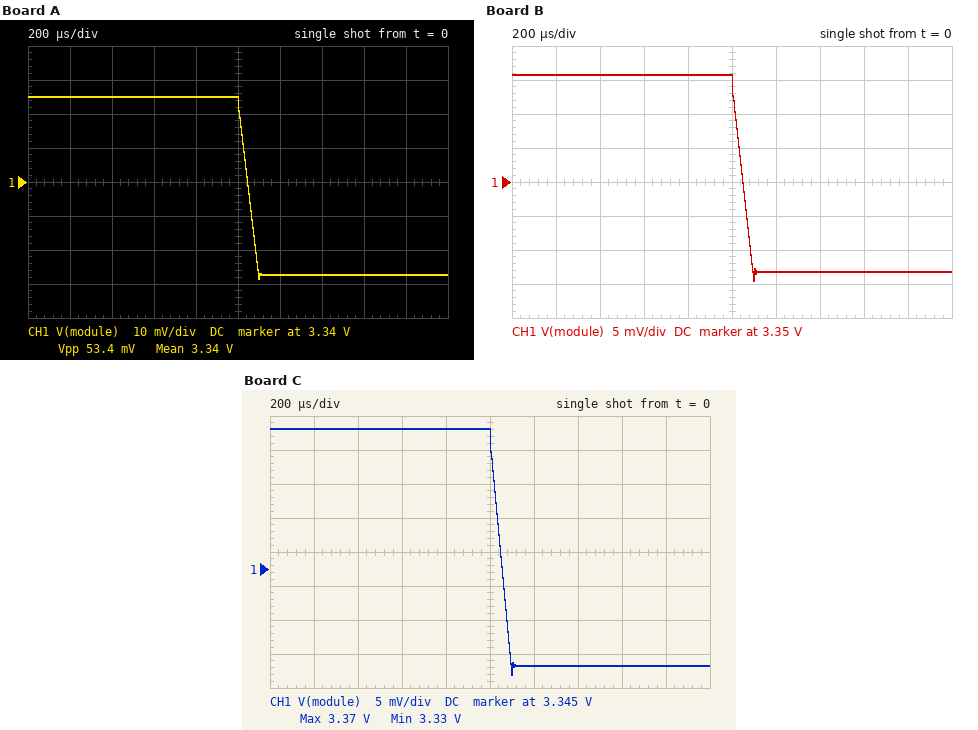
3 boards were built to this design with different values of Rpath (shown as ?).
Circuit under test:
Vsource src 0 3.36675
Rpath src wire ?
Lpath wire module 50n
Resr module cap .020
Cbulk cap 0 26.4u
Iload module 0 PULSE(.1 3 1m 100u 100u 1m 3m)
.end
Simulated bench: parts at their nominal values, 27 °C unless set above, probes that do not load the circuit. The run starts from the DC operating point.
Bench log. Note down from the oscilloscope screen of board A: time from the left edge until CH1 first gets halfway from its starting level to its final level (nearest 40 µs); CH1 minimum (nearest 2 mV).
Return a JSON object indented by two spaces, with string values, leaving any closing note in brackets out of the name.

{
  "time from the left edge until CH1 first gets halfway from its starting level to its final level": "1.04 ms",
  "CH1 minimum": "3.312 V"
}
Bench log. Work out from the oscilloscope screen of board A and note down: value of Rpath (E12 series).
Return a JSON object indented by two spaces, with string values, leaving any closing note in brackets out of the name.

{
  "value of Rpath": "0.018 Ω"
}
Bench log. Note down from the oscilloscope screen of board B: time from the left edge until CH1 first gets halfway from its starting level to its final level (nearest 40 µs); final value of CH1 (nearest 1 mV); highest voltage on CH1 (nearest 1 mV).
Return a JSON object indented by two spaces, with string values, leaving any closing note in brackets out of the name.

{
  "time from the left edge until CH1 first gets halfway from its starting level to its final level": "1.04 ms",
  "final value of CH1": "3.337 V",
  "highest voltage on CH1": "3.366 V"
}
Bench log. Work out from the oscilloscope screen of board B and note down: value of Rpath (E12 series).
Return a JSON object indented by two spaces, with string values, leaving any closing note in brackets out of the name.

{
  "value of Rpath": "0.01 Ω"
}
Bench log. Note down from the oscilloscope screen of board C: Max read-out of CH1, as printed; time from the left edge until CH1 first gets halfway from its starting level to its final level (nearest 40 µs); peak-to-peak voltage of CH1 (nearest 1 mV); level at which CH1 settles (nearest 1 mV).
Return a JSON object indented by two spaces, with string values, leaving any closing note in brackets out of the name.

{
  "Max read-out of CH1, as printed": "3.37 V",
  "time from the left edge until CH1 first gets halfway from its starting level to its final level": "1.04 ms",
  "peak-to-peak voltage of CH1": "36 mV",
  "level at which CH1 settles": "3.331 V"
}
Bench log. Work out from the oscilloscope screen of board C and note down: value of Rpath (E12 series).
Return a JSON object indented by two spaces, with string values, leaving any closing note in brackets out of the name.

{
  "value of Rpath": "0.012 Ω"
}
